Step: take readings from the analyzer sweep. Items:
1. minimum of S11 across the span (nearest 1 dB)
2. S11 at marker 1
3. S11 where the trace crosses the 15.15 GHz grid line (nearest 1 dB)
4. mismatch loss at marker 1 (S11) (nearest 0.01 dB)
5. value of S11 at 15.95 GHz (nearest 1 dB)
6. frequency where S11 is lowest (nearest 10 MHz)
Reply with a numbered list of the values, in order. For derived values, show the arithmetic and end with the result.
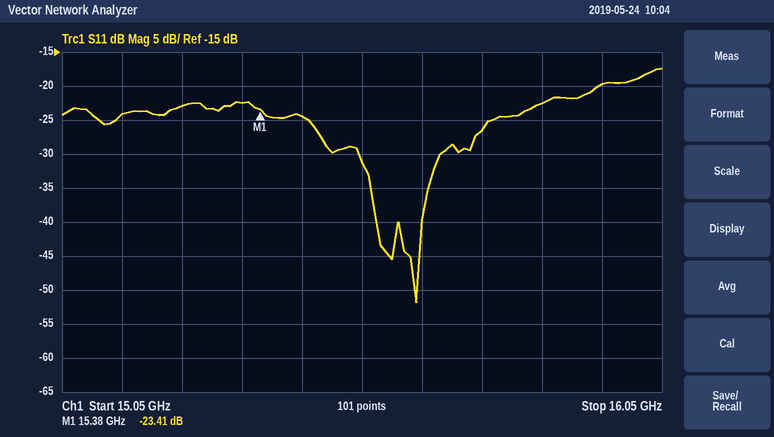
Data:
1. -52 dB
2. -23.41 dB
3. -24 dB
4. −10 log10(1 − 10^(-23.41/10)) ≈ 0.02 dB
5. -20 dB
6. 15.64 GHz
